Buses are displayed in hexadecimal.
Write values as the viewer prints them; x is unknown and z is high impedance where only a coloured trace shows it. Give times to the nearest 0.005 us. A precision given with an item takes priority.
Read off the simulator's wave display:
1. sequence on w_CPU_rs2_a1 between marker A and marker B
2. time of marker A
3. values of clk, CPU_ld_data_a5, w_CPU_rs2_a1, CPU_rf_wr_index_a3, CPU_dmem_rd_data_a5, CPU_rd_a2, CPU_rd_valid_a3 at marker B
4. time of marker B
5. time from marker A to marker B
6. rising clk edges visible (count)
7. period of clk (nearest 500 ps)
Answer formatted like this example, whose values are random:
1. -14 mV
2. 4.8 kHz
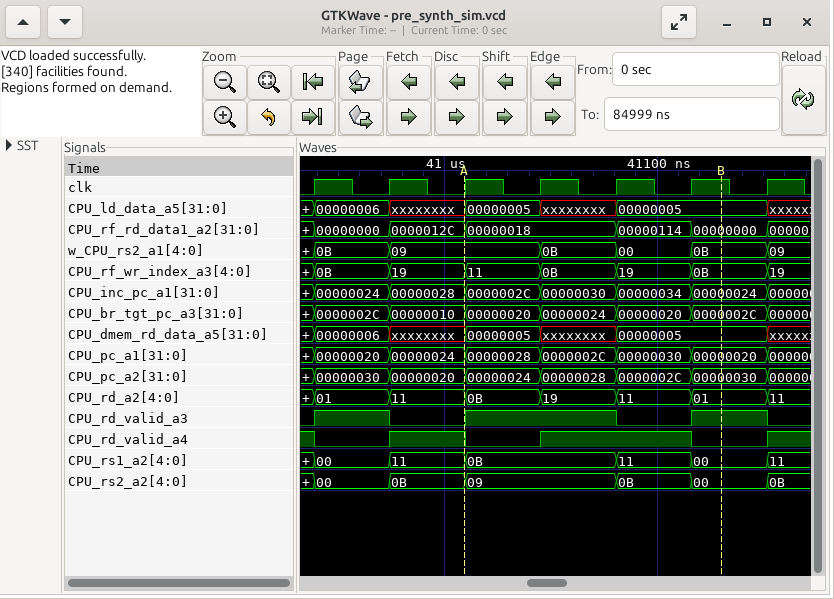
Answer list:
1. 09, 0B, 00, 0B
2. 41.01 us
3. clk=1, CPU_ld_data_a5=00000005, w_CPU_rs2_a1=0B, CPU_rf_wr_index_a3=0B, CPU_dmem_rd_data_a5=00000005, CPU_rd_a2=01, CPU_rd_valid_a3=1
4. 41.13 us
5. 0.12 us
6. 7
7. 35500 ps
